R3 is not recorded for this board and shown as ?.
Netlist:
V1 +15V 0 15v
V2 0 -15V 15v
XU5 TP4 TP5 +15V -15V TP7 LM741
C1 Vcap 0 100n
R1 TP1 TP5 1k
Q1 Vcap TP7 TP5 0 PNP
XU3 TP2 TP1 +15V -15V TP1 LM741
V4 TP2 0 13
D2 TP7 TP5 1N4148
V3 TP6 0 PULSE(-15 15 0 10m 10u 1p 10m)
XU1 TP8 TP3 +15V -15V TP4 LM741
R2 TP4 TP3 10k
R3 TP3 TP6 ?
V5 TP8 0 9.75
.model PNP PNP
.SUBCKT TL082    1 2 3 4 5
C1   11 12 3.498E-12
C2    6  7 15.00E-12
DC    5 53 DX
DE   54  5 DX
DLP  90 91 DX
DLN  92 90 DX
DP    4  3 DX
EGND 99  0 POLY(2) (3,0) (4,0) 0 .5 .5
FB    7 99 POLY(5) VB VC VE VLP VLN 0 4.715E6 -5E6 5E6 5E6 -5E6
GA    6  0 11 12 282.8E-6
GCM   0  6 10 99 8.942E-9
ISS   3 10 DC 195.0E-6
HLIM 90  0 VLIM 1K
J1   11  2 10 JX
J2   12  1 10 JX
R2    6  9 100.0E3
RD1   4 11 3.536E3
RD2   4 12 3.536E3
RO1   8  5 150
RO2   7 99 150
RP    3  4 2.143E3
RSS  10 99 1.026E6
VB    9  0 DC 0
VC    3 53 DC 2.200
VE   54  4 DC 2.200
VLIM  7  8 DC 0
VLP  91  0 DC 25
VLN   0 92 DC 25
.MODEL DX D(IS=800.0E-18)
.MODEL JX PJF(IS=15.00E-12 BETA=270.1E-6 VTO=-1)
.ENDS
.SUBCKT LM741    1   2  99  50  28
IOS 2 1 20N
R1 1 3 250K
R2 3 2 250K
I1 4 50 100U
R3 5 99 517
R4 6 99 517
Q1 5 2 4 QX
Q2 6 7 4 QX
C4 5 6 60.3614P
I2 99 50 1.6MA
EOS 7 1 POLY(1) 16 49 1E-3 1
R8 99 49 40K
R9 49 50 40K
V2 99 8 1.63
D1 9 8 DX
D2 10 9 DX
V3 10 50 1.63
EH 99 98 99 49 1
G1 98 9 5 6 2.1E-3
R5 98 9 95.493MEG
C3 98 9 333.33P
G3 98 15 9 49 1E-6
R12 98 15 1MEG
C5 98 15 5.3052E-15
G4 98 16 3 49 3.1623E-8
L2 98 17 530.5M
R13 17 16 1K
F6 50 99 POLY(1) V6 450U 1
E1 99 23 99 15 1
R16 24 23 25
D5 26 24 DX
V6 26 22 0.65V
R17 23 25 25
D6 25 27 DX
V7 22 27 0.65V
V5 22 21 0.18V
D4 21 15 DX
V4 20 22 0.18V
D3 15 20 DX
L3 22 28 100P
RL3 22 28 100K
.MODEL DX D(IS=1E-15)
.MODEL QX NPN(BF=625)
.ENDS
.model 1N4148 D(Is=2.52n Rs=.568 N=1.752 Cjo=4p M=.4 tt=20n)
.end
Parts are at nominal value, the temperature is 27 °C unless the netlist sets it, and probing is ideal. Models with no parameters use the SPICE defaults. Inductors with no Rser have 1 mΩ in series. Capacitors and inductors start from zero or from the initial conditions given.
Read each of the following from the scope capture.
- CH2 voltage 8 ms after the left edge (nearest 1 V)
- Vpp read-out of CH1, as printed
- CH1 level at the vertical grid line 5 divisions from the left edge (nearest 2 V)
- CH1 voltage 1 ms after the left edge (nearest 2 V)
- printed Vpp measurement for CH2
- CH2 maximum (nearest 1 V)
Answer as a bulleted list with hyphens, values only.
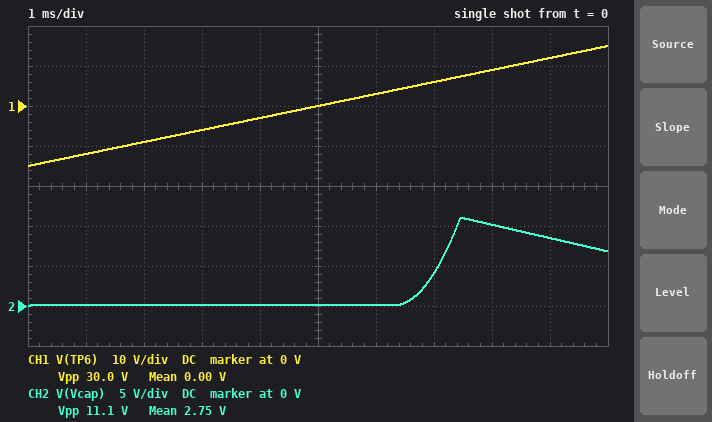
- 10 V
- 30.0 V
- 0 V
- -12 V
- 11.1 V
- 11 V
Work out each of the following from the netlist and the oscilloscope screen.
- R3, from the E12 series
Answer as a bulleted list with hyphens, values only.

- 18 kΩ
